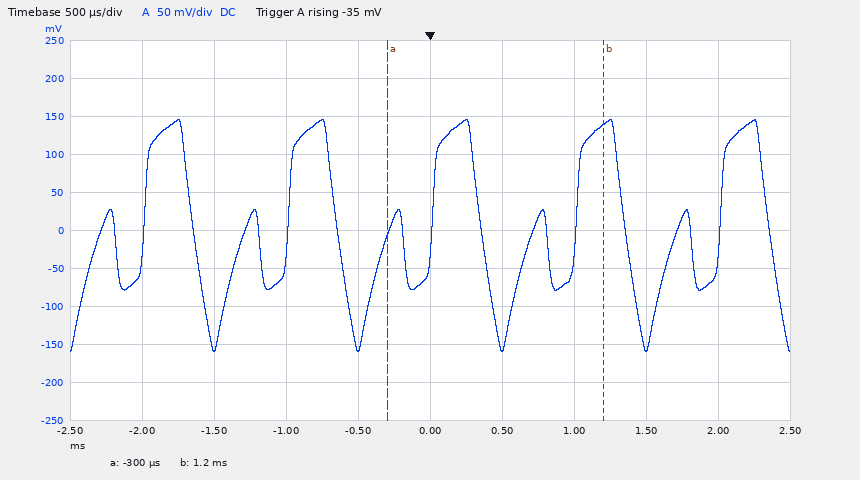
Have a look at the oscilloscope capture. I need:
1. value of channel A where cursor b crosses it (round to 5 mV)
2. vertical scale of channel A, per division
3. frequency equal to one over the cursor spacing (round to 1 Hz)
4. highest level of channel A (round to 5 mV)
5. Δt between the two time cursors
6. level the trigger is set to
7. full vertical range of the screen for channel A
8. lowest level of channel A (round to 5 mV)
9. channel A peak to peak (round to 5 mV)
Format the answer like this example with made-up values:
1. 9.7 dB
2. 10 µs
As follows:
1. 140 mV
2. 50 mV
3. 667 Hz
4. 145 mV
5. 1.50 ms
6. -35 mV
7. 500 mV
8. -160 mV
9. 305 mV
